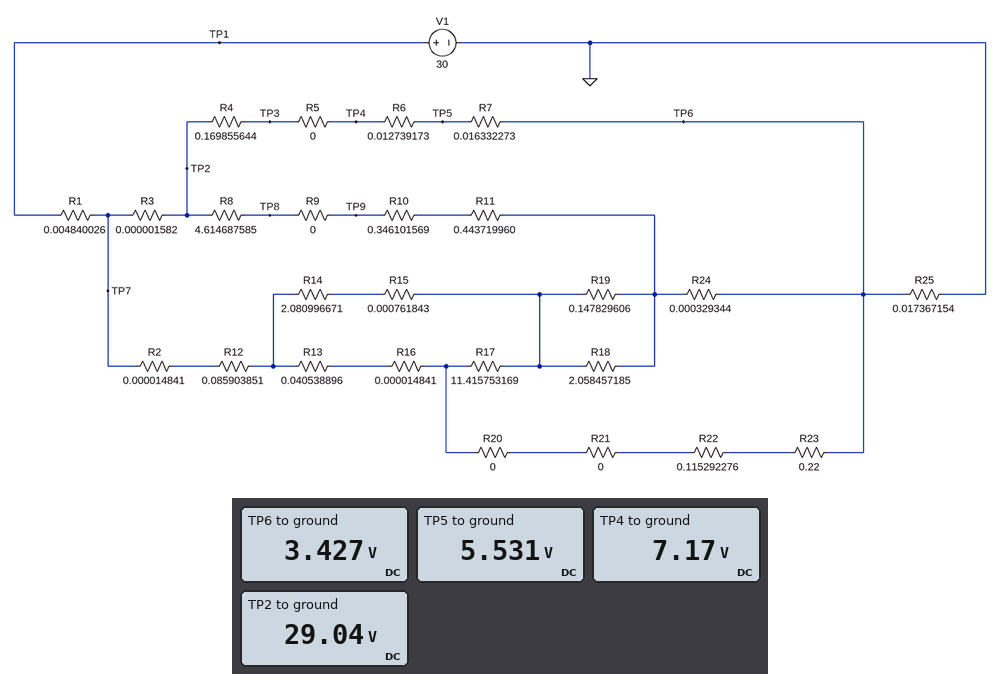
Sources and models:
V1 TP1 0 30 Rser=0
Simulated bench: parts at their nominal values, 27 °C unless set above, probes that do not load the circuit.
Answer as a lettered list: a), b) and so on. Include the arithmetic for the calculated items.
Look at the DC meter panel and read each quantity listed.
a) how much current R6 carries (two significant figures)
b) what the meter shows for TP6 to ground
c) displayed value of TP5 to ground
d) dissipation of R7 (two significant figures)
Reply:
a) (7.17 V - 5.531 V) / 12.74 mΩ = 130 A
b) 3.427 V
c) 5.531 V
d) (5.531 V - 3.427 V)^2 / 16.33 mΩ = 270 W
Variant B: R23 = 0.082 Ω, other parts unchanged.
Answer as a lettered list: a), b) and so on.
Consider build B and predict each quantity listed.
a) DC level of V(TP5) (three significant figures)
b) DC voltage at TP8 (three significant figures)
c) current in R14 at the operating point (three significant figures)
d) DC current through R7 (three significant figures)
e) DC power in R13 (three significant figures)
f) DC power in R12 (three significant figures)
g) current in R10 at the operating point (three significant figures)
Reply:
a) 5.82 V
b) 7.44 V
c) 8.01 A
d) 127 A
e) 237 W
f) 613 W
g) 4.66 A
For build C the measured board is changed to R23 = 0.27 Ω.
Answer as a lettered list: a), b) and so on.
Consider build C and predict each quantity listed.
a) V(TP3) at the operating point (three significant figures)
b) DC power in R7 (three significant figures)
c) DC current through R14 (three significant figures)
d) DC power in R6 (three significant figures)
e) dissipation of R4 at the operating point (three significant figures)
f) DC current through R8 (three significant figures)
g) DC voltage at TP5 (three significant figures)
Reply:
a) 7.11 V
b) 273 W
c) 9.20 A
d) 213 W
e) 2.84 kW
f) 4.76 A
g) 5.46 V
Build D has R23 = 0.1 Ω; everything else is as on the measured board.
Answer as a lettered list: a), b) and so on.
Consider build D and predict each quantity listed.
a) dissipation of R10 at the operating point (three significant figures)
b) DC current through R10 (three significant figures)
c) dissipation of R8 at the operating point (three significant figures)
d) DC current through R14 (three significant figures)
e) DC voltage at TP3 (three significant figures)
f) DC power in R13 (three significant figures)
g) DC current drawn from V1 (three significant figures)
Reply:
a) 7.57 W
b) 4.68 A
c) 101 W
d) 8.18 A
e) 7.39 V
f) 214 W
g) 213 A
